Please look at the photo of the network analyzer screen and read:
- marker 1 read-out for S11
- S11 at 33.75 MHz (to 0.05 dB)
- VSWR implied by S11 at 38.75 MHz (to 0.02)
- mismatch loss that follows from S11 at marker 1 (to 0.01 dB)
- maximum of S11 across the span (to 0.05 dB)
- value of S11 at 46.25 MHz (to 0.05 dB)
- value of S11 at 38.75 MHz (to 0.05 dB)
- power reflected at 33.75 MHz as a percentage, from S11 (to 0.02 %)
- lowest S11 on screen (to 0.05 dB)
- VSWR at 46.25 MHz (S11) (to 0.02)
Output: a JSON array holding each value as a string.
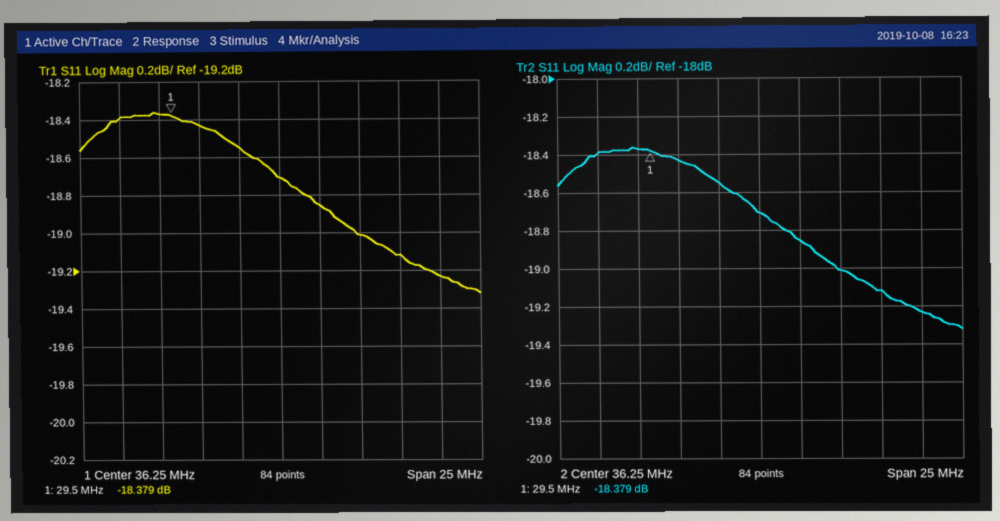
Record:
["-18.379 dB", "-18.55 dB", "1.26", "0.06 dB", "-18.35 dB", "-19.25 dB", "-18.85 dB", "1.40 %", "-19.30 dB", "1.24"]
